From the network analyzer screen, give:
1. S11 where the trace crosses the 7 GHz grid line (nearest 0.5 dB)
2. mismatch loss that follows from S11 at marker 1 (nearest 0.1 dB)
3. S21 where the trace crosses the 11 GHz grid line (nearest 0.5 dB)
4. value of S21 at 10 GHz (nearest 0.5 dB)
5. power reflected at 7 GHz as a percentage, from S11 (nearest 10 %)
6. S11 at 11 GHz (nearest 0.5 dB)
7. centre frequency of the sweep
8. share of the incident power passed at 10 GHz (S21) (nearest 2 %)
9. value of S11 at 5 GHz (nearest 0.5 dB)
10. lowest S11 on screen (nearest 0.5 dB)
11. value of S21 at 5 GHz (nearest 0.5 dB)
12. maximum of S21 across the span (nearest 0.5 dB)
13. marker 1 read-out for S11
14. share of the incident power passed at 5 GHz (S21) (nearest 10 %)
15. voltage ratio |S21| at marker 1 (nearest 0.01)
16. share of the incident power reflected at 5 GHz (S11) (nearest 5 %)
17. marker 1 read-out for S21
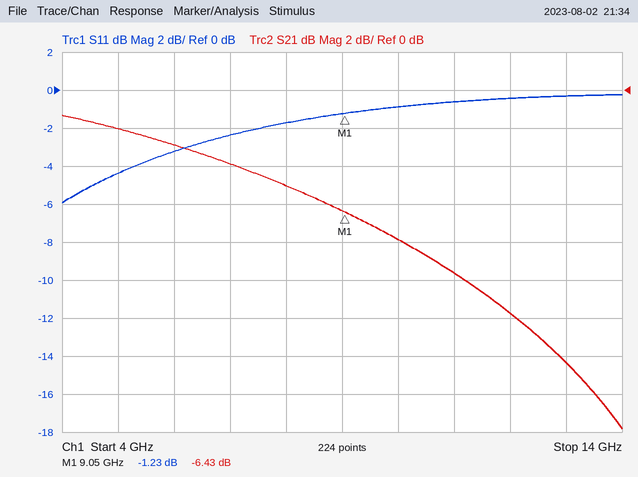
-2.5 dB
6.1 dB
-9.5 dB
-8.0 dB
60 %
-0.5 dB
9 GHz
16 %
-4.5 dB
-6.0 dB
-2.0 dB
-1.5 dB
-1.23 dB
60 %
0.48
35 %
-6.43 dB
